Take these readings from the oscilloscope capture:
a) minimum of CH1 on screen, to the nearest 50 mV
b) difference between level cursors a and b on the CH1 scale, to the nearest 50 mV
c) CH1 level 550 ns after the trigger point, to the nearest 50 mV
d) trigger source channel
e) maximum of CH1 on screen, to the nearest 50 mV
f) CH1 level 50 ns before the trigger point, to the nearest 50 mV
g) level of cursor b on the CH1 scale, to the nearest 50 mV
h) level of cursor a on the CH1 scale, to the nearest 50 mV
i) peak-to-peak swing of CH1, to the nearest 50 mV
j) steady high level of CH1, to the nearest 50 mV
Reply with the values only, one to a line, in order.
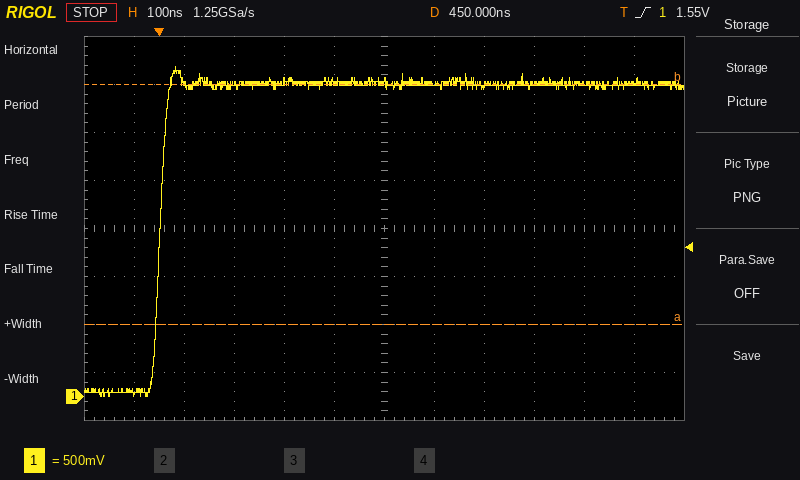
0 mV
2.50 V
3.25 V
CH1
3.45 V
50 mV
3.25 V
750 mV
3.45 V
3.25 V
